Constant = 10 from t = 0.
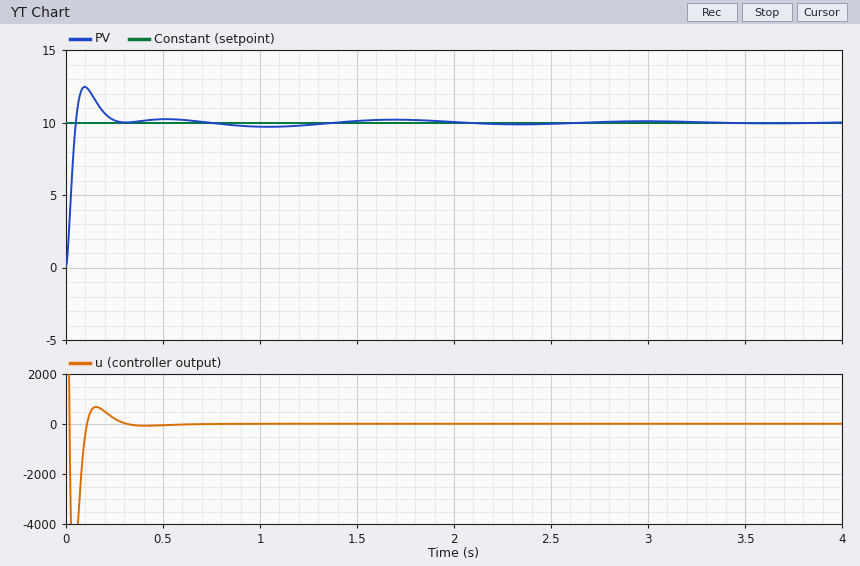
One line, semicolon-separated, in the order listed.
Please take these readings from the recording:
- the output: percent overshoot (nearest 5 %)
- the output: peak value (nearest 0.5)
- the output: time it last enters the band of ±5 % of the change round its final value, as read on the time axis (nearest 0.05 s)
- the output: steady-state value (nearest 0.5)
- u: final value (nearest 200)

25 %; 12.5; 0.20 s; 10.0; 0
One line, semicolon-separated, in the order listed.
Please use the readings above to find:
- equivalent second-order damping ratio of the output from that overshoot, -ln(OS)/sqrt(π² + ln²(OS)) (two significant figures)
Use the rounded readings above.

0.40
